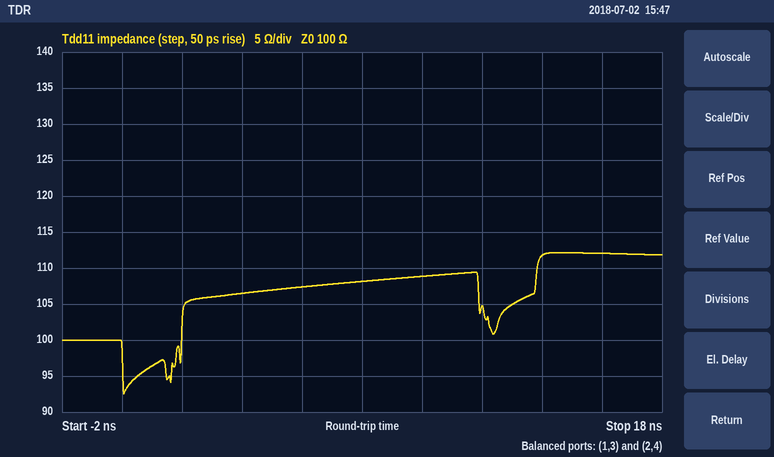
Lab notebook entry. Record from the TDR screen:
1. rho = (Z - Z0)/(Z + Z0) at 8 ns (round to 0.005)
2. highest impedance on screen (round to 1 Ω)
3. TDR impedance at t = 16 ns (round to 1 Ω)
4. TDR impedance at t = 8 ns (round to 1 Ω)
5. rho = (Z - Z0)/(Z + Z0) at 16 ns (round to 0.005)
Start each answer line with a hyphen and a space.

- +0.040
- 112 Ω
- 112 Ω
- 108 Ω
- +0.055
